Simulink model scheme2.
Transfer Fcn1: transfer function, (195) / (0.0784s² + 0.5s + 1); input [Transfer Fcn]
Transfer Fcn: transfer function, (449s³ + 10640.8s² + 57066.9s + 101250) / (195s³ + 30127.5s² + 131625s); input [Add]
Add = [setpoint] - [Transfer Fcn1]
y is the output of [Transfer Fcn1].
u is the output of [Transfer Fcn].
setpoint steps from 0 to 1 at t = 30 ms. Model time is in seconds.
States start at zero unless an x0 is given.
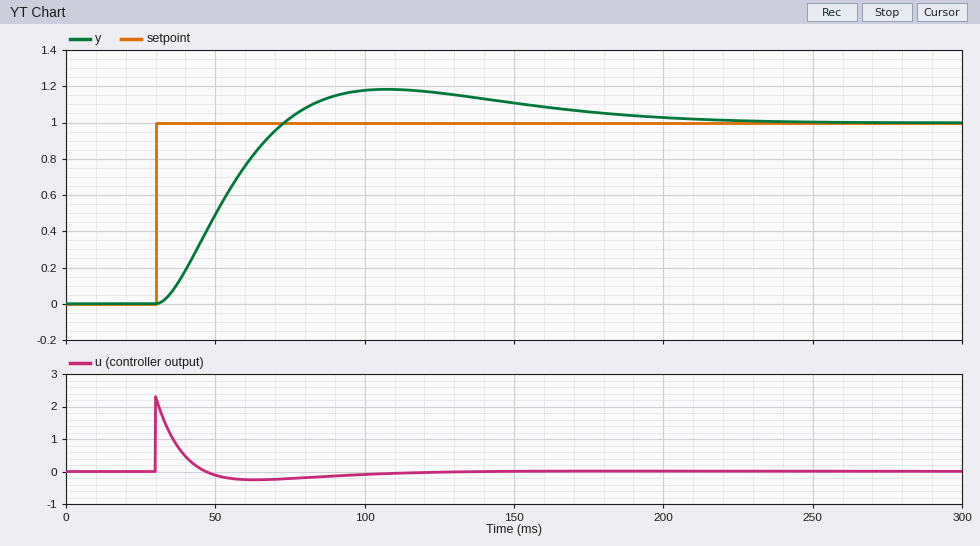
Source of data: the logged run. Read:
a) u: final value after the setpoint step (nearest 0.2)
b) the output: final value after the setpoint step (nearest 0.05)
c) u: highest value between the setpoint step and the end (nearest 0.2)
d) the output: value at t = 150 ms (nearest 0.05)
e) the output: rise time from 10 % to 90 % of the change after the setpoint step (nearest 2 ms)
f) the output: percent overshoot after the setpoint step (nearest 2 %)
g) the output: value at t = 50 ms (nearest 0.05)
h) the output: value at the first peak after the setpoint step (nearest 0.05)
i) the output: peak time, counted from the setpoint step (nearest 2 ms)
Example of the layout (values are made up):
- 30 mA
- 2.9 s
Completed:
- 0.0
- 1.00
- 2.2
- 1.10
- 30 ms
- 18 %
- 0.50
- 1.20
- 78 ms
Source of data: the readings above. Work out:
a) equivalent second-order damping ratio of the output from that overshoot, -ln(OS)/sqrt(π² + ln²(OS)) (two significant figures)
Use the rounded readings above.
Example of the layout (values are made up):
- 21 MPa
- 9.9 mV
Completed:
- 0.48
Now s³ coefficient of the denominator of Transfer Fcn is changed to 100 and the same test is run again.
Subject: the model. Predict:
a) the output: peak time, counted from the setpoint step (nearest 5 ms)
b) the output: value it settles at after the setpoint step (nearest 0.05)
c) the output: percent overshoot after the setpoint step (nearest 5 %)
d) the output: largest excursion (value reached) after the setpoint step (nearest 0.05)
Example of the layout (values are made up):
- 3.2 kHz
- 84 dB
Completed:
- 85 ms
- 1.00
- 15 %
- 1.15
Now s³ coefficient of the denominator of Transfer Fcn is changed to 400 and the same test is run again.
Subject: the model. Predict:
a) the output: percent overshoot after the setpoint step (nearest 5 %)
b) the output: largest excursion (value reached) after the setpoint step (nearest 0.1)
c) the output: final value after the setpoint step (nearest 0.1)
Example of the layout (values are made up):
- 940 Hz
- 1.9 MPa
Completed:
- 30 %
- 1.3
- 1.0
